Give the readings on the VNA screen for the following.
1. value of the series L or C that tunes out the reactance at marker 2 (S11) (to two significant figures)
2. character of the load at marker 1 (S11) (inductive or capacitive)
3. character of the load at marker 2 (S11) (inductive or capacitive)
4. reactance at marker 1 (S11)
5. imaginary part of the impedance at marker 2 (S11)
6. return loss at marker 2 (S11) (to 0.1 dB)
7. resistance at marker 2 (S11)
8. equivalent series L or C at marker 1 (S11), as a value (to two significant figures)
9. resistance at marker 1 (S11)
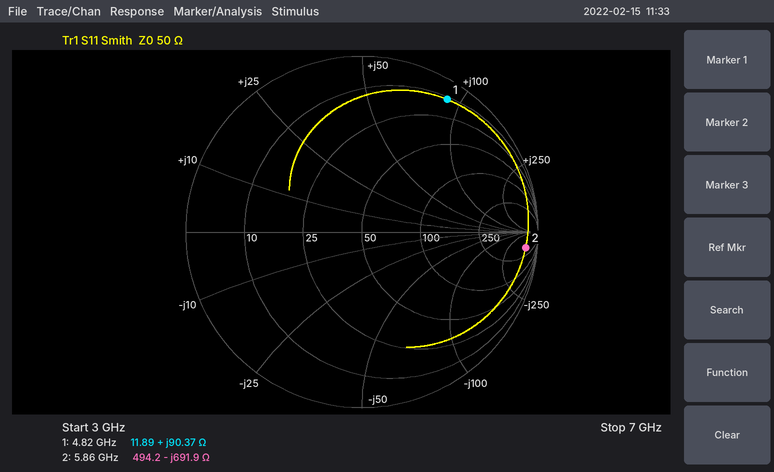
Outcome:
19 nH
inductive
capacitive
+90.37 Ω
-691.9 Ω
0.6 dB
494.2 Ω
3.0 nH
11.89 Ω
